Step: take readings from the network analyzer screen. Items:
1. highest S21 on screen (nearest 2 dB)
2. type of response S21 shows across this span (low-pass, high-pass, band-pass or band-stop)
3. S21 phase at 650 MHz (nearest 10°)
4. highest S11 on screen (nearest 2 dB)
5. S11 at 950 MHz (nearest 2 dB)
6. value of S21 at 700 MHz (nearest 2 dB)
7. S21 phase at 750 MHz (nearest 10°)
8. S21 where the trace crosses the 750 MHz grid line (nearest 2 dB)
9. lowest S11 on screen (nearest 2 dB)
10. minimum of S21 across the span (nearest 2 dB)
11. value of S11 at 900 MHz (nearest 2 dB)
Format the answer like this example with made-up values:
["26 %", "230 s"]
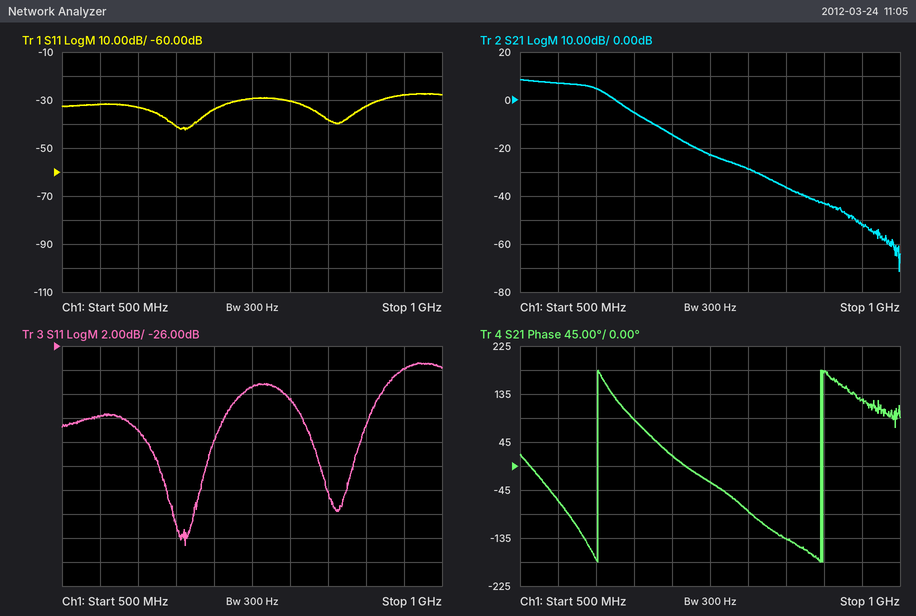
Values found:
["8 dB", "low-pass", "90°", "-28 dB", "-28 dB", "-14 dB", "-30°", "-22 dB", "-42 dB", "-72 dB", "-32 dB"]
